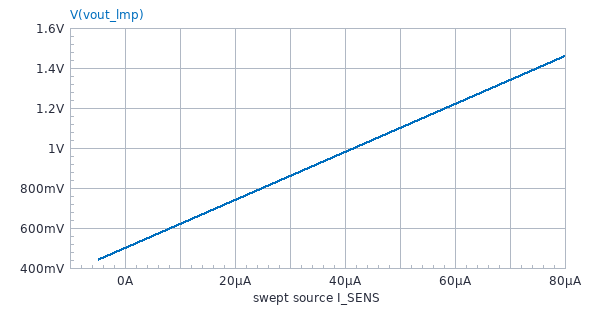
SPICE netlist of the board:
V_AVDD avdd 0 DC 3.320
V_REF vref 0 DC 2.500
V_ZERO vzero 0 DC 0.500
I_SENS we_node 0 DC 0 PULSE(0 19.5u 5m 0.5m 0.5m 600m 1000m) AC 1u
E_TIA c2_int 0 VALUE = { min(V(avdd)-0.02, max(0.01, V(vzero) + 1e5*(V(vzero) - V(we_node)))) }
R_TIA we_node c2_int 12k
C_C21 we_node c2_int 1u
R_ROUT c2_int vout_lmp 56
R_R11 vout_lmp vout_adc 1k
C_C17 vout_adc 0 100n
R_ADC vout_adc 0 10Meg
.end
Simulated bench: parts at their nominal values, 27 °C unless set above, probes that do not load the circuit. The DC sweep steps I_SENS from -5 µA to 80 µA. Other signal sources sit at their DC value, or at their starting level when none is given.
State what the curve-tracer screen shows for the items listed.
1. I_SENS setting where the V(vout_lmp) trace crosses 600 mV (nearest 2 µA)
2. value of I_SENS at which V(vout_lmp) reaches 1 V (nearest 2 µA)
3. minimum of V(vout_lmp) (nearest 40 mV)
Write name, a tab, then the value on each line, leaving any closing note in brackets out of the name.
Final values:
I_SENS setting where the V(vout_lmp) trace crosses 600 mV	8 µA
value of I_SENS at which V(vout_lmp) reaches 1 V	42 µA
minimum of V(vout_lmp)	440 mV
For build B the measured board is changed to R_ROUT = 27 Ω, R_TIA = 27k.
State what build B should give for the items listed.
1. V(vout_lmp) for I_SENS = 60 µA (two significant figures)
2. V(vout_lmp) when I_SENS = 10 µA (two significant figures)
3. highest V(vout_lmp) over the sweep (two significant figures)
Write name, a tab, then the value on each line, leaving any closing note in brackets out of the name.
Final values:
V(vout_lmp) for I_SENS = 60 µA	2.1 V
V(vout_lmp) when I_SENS = 10 µA	770 mV
highest V(vout_lmp) over the sweep	2.7 V
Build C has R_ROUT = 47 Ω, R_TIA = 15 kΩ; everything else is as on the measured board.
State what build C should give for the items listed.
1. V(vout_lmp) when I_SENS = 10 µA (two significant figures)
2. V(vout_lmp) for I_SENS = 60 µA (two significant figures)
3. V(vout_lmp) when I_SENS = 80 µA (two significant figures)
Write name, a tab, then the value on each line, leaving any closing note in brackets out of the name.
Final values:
V(vout_lmp) when I_SENS = 10 µA	650 mV
V(vout_lmp) for I_SENS = 60 µA	1.4 V
V(vout_lmp) when I_SENS = 80 µA	1.7 V
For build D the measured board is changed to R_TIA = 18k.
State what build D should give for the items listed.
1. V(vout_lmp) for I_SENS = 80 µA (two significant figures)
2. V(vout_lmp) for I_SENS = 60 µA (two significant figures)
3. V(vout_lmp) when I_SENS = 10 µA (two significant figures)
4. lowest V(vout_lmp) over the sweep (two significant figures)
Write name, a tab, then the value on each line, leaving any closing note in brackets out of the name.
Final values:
V(vout_lmp) for I_SENS = 80 µA	1.9 V
V(vout_lmp) for I_SENS = 60 µA	1.6 V
V(vout_lmp) when I_SENS = 10 µA	680 mV
lowest V(vout_lmp) over the sweep	410 mV
